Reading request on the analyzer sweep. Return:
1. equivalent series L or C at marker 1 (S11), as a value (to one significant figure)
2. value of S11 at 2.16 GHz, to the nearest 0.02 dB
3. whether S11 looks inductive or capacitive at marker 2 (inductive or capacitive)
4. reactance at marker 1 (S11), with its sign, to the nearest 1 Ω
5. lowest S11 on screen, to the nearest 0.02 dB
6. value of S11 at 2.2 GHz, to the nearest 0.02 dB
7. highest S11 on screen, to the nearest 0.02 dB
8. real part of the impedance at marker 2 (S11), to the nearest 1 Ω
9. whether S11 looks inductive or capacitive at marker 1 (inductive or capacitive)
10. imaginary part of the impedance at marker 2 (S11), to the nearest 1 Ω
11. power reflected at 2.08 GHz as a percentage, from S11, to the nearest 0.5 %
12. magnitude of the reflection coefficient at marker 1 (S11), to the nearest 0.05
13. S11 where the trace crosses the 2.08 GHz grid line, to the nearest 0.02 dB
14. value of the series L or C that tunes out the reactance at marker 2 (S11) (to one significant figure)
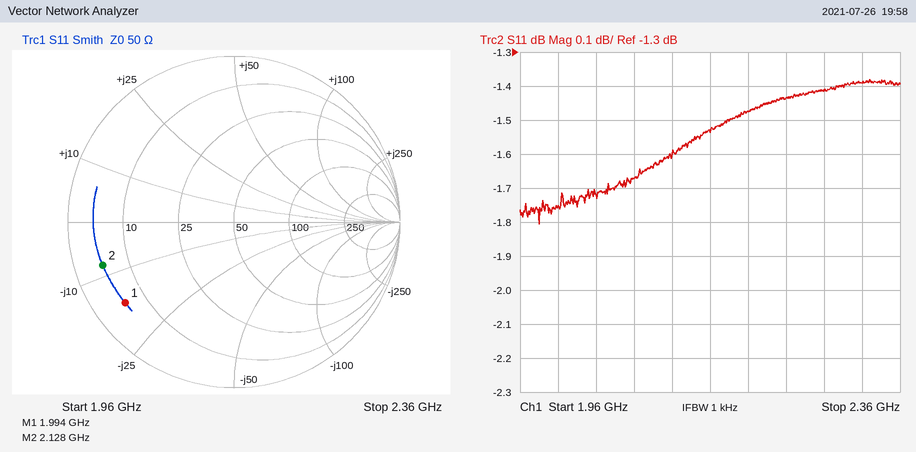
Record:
5 pF
-1.54 dB
capacitive
-16 Ω
-1.80 dB
-1.48 dB
-1.38 dB
5 Ω
capacitive
-8 Ω
68.0 %
0.80
-1.68 dB
600 pH
